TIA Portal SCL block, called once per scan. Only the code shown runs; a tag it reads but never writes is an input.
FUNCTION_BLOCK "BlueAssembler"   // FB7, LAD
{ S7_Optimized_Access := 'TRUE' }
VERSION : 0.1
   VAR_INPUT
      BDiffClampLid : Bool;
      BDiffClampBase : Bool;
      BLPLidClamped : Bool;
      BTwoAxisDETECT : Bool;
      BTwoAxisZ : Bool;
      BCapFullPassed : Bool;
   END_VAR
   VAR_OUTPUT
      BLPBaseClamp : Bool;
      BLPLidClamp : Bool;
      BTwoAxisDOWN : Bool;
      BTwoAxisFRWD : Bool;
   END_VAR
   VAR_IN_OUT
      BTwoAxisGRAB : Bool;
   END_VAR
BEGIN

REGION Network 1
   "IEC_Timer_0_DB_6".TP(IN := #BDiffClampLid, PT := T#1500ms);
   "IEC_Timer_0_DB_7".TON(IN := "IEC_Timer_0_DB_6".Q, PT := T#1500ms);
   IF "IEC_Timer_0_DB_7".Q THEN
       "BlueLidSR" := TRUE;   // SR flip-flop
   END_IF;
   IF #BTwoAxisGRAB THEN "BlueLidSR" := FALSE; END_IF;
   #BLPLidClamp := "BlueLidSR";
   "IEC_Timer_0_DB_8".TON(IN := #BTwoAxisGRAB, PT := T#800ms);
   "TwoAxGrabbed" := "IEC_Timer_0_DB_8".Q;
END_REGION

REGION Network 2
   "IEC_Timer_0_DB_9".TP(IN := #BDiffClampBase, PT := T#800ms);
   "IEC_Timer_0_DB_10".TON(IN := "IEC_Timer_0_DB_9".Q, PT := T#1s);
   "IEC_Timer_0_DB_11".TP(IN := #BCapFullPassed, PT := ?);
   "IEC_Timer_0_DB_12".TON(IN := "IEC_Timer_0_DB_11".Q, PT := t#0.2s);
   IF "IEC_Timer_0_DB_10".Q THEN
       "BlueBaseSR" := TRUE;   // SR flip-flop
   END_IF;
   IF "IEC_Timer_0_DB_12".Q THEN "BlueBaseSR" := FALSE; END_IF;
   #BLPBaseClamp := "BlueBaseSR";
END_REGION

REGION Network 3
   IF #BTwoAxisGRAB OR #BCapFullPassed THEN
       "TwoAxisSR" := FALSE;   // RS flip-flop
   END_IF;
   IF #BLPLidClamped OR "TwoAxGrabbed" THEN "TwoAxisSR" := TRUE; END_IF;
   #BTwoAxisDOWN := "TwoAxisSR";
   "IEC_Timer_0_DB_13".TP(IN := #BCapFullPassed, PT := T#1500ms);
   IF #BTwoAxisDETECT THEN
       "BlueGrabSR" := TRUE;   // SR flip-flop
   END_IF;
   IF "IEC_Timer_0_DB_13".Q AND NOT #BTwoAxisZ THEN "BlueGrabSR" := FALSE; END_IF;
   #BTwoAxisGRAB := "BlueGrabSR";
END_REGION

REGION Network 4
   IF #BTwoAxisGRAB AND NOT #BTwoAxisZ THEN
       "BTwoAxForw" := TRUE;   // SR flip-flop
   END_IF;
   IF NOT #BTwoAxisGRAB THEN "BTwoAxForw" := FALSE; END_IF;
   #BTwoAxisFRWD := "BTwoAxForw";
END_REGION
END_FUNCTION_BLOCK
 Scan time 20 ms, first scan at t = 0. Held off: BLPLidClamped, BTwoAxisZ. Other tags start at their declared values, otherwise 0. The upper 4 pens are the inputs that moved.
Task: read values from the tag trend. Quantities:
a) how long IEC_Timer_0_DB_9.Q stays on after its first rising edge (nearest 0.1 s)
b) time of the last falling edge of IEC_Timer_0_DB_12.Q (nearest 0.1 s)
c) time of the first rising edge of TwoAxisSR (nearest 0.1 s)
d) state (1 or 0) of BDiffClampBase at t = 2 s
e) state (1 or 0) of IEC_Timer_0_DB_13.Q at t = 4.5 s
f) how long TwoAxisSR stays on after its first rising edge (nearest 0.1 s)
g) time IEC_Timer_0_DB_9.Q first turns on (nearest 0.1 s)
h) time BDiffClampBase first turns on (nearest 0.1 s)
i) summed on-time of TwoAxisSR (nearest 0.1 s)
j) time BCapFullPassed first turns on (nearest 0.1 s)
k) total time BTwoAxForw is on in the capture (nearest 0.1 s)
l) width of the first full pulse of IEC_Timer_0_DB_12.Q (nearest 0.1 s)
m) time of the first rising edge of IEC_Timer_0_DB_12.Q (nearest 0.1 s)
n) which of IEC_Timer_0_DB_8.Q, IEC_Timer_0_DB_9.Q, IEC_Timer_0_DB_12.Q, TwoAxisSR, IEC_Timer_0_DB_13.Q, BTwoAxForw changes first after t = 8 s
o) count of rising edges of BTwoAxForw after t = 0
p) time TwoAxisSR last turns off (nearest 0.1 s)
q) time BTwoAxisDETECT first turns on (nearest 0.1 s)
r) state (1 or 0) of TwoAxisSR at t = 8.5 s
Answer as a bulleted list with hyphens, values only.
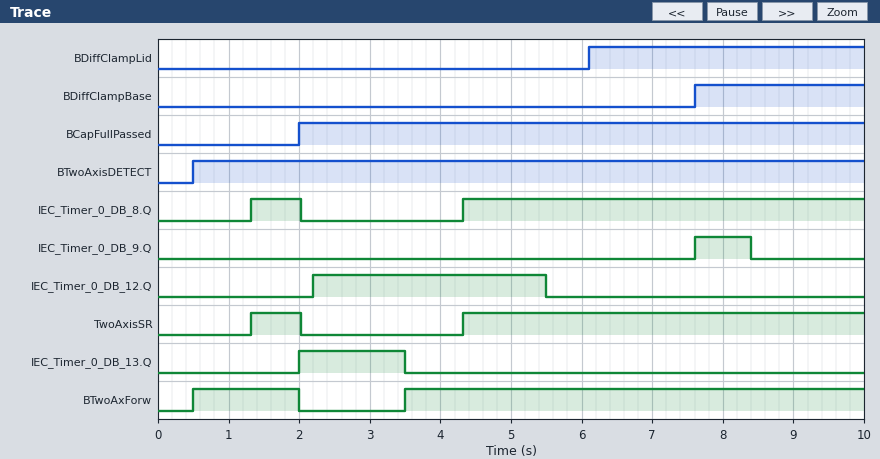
- 0.8 s
- 5.5 s
- 1.3 s
- 0
- 0
- 0.7 s
- 7.6 s
- 7.6 s
- 6.4 s
- 2.0 s
- 8.0 s
- 3.3 s
- 2.2 s
- IEC_Timer_0_DB_9.Q
- 2
- 2.0 s
- 0.5 s
- 1
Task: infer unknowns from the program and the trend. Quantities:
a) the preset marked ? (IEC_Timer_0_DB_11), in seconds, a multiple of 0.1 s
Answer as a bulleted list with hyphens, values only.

- 3.5 s
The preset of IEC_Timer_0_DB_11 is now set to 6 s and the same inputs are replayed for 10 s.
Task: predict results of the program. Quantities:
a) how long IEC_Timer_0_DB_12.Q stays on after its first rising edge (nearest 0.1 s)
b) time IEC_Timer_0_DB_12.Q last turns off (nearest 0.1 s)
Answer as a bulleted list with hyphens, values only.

- 5.8 s
- 8.0 s
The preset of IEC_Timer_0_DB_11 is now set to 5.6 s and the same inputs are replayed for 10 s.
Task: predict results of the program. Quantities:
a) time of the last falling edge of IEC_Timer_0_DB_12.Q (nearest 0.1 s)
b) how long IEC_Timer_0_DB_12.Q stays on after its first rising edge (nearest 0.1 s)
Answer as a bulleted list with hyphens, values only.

- 7.6 s
- 5.4 s
